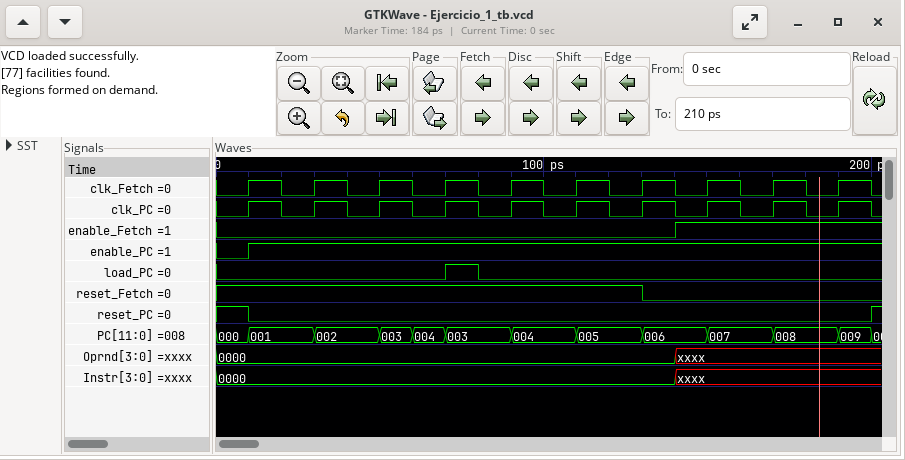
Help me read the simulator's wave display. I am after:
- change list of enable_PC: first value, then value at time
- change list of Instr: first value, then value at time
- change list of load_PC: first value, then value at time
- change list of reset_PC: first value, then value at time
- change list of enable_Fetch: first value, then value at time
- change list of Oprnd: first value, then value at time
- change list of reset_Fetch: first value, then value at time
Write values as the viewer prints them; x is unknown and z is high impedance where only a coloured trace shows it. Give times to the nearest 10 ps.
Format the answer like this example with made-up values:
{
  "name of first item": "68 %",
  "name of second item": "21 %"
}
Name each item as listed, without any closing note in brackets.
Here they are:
{
  "change list of enable_PC: first value, then value at time": "0, 1 at 10 ps",
  "change list of Instr: first value, then value at time": "0000, xxxx at 140 ps",
  "change list of load_PC: first value, then value at time": "0, 1 at 70 ps, 0 at 80 ps",
  "change list of reset_PC: first value, then value at time": "1, 0 at 10 ps, 1 at 200 ps",
  "change list of enable_Fetch: first value, then value at time": "0, 1 at 140 ps",
  "change list of Oprnd: first value, then value at time": "0000, xxxx at 140 ps",
  "change list of reset_Fetch: first value, then value at time": "1, 0 at 130 ps"
}
